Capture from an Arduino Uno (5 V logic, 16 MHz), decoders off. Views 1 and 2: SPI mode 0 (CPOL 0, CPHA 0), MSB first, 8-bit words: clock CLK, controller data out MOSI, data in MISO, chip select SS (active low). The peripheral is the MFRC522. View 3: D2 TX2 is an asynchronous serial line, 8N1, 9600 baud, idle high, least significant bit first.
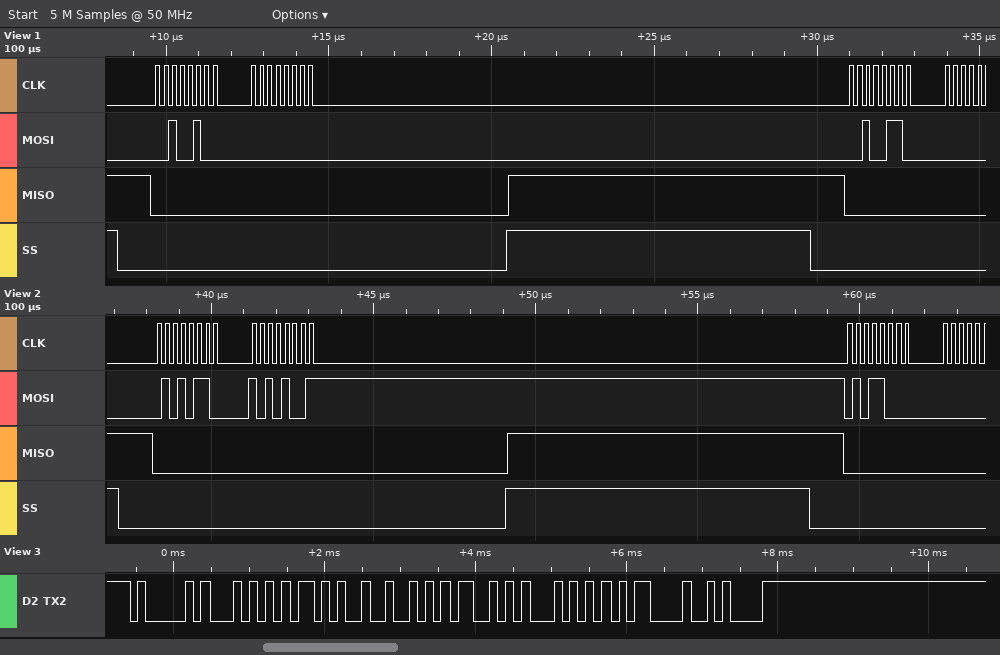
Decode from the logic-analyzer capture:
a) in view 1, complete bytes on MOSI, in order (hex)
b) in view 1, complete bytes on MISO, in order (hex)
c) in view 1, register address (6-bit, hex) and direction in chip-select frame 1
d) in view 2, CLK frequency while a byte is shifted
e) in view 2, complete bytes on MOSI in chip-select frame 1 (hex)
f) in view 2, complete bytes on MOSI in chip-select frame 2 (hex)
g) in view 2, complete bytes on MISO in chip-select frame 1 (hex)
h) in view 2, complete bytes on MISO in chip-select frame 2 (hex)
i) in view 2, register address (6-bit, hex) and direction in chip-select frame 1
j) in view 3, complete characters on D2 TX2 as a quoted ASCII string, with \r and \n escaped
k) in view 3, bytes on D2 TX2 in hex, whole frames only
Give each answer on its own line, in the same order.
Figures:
24 00 26
00 00 00
0x12 write
4 MHz
0x56 0xA9
0x58
0x00 0x00
0x00
0x2B write
"AT+RST\r\n"
41 54 2B 52 53 54 0D 0A
